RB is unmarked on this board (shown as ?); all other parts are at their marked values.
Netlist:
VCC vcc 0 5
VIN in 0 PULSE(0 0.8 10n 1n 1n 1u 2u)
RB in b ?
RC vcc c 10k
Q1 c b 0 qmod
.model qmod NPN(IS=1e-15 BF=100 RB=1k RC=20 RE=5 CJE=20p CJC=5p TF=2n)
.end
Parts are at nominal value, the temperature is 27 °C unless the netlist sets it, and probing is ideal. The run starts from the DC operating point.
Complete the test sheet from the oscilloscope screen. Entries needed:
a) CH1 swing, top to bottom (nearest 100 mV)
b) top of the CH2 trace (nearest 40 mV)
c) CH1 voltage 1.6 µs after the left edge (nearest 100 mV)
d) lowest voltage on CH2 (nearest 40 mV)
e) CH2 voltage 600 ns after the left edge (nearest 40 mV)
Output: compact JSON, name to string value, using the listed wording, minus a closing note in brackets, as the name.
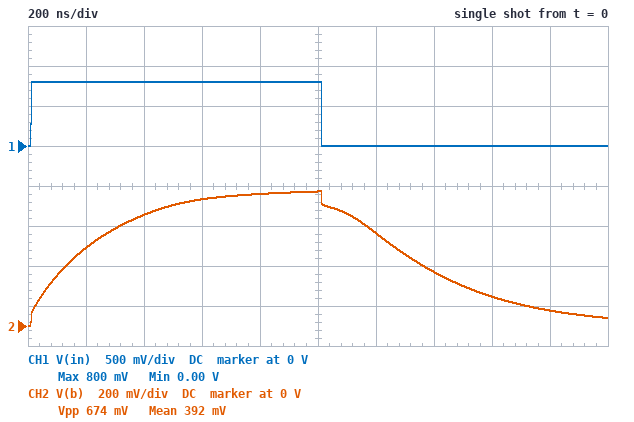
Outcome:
{"CH1 swing, top to bottom": "800 mV", "top of the CH2 trace": "680 mV", "CH1 voltage 1.6 µs after the left edge": "0 V", "lowest voltage on CH2": "0 V", "CH2 voltage 600 ns after the left edge": "640 mV"}
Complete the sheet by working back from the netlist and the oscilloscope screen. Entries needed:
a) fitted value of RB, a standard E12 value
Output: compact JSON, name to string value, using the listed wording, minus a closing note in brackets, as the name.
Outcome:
{"fitted value of RB, a standard E12 value": "12 kΩ"}
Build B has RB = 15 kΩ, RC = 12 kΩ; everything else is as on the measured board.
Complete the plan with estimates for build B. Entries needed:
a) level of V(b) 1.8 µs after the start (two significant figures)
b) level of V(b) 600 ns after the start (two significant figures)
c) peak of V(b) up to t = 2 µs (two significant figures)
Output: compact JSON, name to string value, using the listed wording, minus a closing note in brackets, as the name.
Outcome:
{"level of V(b) 1.8 µs after the start": "110 mV", "level of V(b) 600 ns after the start": "600 mV", "peak of V(b) up to t = 2 µs": "660 mV"}
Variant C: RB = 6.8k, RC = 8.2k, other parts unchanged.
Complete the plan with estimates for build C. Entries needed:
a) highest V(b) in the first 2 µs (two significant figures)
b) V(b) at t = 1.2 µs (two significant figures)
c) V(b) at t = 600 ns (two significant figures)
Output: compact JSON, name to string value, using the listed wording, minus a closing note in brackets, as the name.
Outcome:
{"highest V(b) in the first 2 µs": "700 mV", "V(b) at t = 1.2 µs": "410 mV", "V(b) at t = 600 ns": "680 mV"}
